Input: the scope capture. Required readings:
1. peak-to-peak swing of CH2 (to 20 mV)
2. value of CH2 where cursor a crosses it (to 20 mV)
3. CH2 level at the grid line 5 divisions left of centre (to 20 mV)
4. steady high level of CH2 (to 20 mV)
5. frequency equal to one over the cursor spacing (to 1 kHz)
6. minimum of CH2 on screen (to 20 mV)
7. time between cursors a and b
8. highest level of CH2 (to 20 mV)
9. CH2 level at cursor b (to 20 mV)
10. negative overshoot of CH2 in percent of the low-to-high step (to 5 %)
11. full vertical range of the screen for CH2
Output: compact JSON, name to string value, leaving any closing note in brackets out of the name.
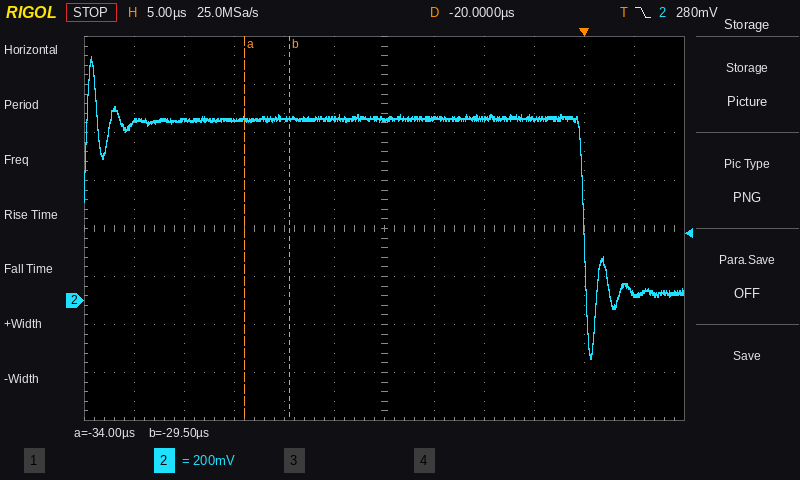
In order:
{"peak-to-peak swing of CH2": "1.26 V", "value of CH2 where cursor a crosses it": "760 mV", "CH2 level at the grid line 5 divisions left of centre": "740 mV", "steady high level of CH2": "760 mV", "frequency equal to one over the cursor spacing": "222 kHz", "minimum of CH2 on screen": "-240 mV", "time between cursors a and b": "4.5 µs", "highest level of CH2": "1.02 V", "CH2 level at cursor b": "760 mV", "negative overshoot of CH2 in percent of the low-to-high step": "35 %", "full vertical range of the screen for CH2": "1.6 V"}
